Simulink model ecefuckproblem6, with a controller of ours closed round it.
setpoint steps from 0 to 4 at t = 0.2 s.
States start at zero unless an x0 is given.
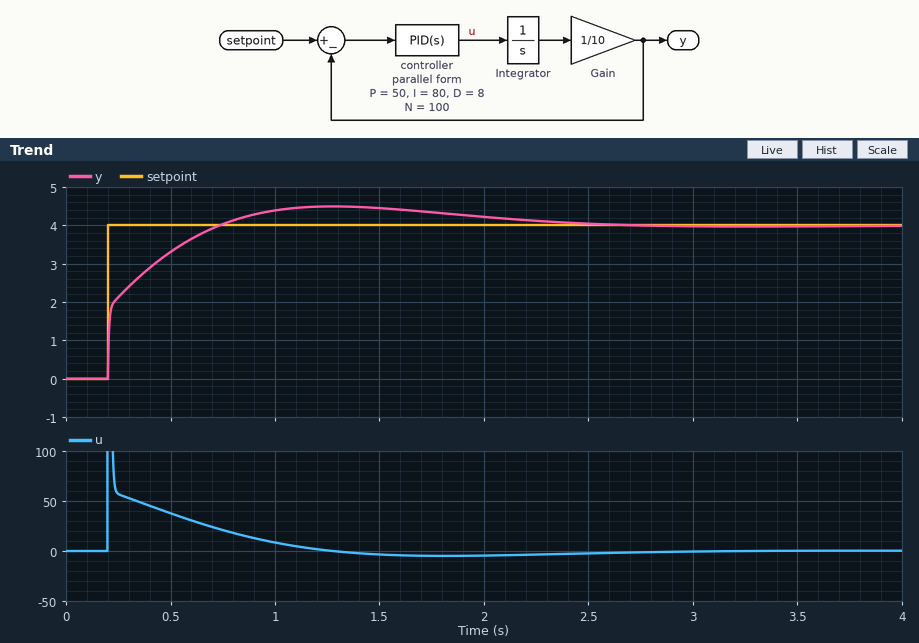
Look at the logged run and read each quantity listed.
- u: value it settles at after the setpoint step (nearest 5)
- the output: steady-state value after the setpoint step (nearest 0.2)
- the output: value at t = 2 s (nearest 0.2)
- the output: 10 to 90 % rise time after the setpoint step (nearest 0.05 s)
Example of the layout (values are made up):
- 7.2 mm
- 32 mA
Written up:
- 0
- 4.0
- 4.2
- 0.40 s
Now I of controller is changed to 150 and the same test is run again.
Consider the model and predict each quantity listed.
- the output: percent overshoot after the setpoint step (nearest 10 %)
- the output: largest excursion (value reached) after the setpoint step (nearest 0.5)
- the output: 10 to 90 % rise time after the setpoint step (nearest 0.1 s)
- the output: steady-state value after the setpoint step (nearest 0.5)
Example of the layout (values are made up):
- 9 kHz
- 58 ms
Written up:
- 20 %
- 4.5
- 0.3 s
- 4.0
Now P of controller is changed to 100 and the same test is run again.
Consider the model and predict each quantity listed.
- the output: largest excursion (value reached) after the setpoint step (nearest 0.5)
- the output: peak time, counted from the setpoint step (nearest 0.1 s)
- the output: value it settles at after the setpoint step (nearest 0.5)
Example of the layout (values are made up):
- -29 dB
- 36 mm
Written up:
- 4.0
- 0.9 s
- 4.0
